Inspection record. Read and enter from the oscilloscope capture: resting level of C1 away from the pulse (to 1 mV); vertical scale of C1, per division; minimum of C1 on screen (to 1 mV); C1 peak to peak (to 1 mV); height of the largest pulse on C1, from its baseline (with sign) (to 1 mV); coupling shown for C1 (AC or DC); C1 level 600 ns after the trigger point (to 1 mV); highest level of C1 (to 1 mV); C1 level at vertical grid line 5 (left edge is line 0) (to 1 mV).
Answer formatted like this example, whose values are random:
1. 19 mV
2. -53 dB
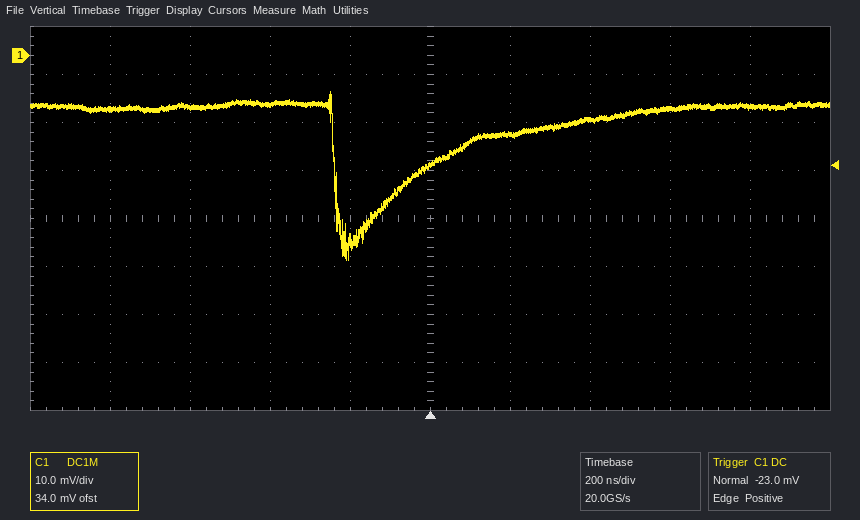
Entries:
1. -11 mV
2. 10 mV
3. -43 mV
4. 35 mV
5. -32 mV
6. DC
7. -11 mV
8. -8 mV
9. -23 mV
